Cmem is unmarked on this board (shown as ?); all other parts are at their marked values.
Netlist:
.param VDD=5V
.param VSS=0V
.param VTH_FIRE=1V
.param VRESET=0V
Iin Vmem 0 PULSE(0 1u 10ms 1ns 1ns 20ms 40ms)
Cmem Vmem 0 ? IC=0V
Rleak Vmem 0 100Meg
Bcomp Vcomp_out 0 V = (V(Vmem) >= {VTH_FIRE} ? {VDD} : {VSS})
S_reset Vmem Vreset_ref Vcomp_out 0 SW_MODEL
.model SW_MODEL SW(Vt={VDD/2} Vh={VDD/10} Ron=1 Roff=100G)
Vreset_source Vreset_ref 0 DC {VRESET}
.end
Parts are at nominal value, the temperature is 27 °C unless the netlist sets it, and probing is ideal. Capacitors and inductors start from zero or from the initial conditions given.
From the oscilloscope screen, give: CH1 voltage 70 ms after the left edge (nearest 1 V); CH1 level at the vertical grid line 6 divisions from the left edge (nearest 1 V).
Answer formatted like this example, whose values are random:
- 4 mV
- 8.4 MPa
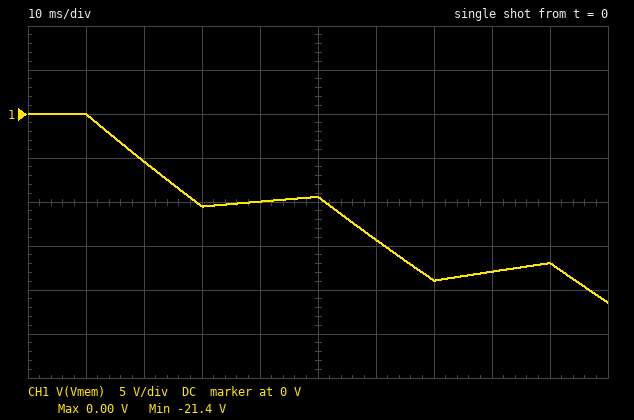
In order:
- -19 V
- -14 V
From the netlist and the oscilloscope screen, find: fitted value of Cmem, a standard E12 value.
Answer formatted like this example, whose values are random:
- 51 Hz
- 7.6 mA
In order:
- 1.8 nF
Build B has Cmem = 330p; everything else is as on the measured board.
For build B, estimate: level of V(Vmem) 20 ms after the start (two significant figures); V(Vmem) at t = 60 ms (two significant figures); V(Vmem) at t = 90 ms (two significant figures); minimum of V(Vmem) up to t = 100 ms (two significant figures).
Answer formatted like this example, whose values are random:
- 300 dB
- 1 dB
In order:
- -26 V
- -44 V
- -32 V
- -59 V
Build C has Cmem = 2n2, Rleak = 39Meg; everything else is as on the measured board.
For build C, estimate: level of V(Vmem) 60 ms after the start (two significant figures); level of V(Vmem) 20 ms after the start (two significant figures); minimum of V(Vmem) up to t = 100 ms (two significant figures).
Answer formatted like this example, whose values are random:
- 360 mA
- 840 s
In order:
- -10 V
- -4.3 V
- -14 V
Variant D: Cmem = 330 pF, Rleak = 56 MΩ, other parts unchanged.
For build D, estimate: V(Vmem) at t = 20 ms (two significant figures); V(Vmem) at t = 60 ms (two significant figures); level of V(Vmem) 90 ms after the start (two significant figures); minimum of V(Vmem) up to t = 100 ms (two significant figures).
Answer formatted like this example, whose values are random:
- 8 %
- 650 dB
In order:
- -23 V
- -31 V
- -14 V
- -41 V
